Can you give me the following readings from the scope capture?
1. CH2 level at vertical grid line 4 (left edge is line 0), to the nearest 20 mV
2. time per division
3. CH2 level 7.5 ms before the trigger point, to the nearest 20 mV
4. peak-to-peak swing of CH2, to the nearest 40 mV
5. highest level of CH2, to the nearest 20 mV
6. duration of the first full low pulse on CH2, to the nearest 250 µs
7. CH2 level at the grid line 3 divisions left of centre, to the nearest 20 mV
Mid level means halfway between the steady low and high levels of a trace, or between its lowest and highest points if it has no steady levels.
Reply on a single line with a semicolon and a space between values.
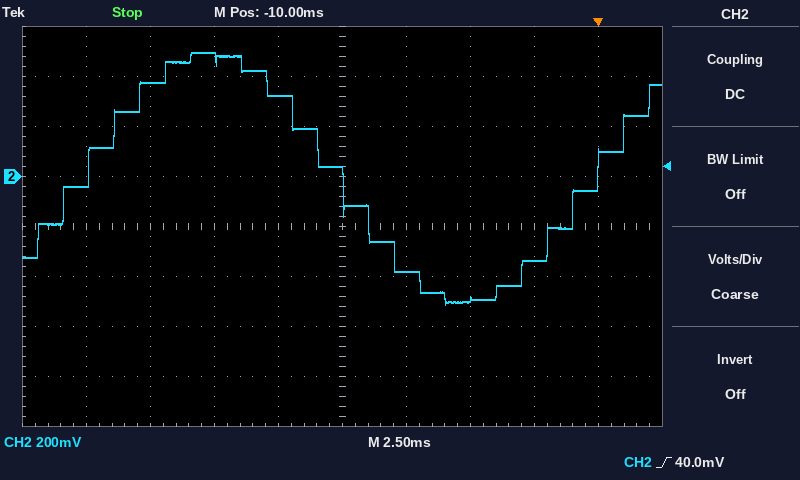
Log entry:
320 mV; 2.5 ms; -380 mV; 1.00 V; 500 mV; 10.00 ms; 380 mV
